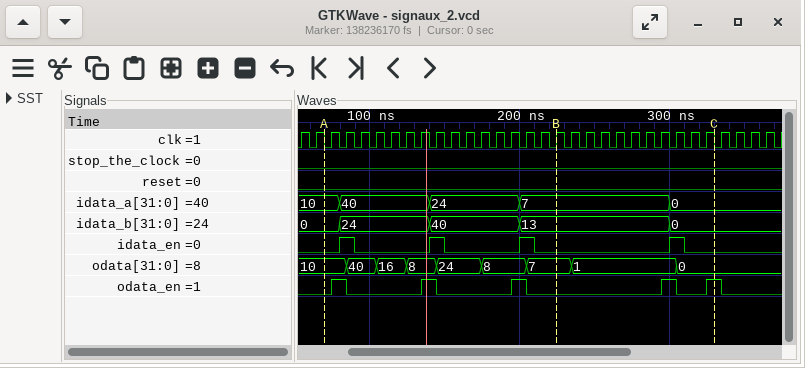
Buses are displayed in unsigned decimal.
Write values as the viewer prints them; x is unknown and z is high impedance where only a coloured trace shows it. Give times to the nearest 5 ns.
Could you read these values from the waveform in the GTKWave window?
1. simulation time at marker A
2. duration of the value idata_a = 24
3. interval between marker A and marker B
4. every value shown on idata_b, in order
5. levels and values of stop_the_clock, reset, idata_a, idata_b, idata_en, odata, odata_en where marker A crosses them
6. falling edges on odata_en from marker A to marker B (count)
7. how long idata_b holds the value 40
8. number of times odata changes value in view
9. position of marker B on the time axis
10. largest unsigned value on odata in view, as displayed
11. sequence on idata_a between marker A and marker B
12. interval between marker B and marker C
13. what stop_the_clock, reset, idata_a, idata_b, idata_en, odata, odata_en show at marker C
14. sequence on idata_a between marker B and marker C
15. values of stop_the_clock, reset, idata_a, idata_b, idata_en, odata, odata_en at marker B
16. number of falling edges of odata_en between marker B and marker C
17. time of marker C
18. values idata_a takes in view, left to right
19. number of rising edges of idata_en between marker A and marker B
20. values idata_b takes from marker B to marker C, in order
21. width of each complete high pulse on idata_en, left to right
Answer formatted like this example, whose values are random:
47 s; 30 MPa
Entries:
70 ns; 60 ns; 155 ns; 0, 24, 40, 13, 0; stop_the_clock=0, reset=0, idata_a=10, idata_b=0, idata_en=0, odata=10, odata_en=0; 3; 60 ns; 8; 225 ns; 40; 10, 40, 24, 7; 105 ns; stop_the_clock=0, reset=0, idata_a=0, idata_b=0, idata_en=0, odata=0, odata_en=1; 7, 0; stop_the_clock=0, reset=0, idata_a=7, idata_b=13, idata_en=0, odata=7, odata_en=0; 1; 330 ns; 10, 40, 24, 7, 0; 3; 13, 0; 10 ns, 10 ns, 10 ns, 10 ns
